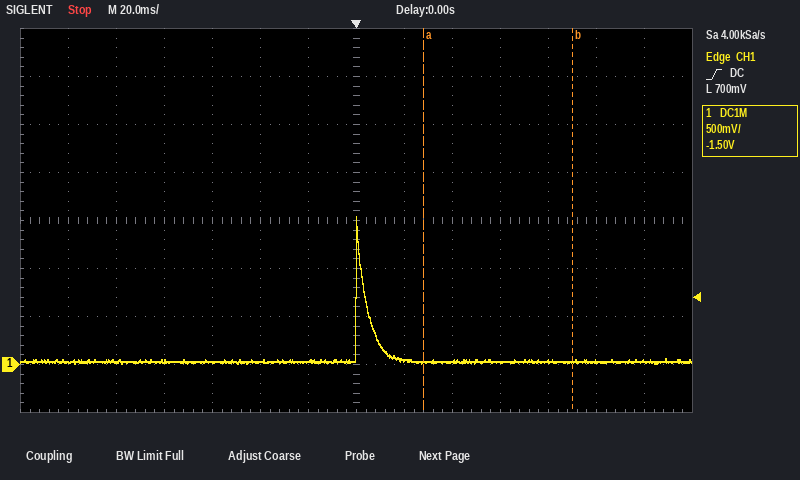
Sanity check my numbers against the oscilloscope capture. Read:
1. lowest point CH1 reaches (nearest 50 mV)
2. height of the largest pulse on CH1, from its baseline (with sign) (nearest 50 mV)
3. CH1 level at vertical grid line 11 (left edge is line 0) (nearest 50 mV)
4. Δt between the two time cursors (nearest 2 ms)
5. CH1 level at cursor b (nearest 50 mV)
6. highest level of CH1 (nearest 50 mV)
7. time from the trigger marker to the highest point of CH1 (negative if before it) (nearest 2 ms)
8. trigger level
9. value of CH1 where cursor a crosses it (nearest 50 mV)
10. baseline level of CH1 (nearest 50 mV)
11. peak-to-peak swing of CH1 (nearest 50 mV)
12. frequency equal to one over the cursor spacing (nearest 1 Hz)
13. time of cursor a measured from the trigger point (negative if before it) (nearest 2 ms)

0 mV
+1.50 V
50 mV
62 ms
50 mV
1.55 V
0 ms
700 mV
0 mV
50 mV
1.55 V
16 Hz
+28 ms
